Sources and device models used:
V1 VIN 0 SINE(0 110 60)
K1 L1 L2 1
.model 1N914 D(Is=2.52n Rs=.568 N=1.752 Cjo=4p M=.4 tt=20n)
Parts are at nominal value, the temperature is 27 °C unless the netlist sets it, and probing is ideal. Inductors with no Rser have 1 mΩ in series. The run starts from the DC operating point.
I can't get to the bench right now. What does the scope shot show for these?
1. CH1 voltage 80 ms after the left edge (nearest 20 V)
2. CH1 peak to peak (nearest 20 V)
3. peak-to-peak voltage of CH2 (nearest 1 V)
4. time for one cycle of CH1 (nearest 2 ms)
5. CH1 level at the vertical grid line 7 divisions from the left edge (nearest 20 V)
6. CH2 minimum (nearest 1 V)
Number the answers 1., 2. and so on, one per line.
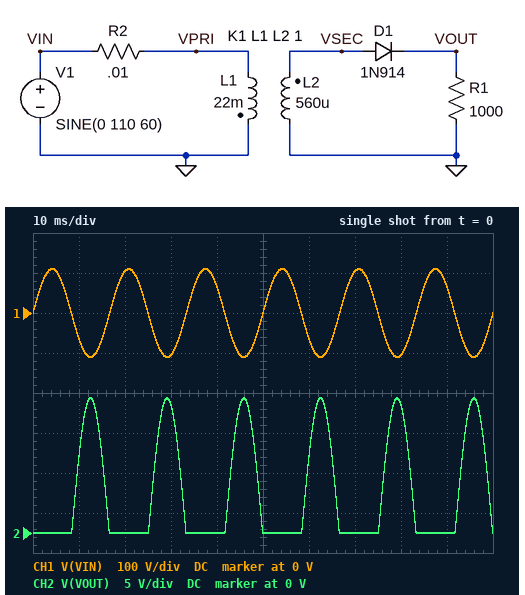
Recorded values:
1. -100 V
2. 220 V
3. 17 V
4. 16 ms
5. 100 V
6. 0 V
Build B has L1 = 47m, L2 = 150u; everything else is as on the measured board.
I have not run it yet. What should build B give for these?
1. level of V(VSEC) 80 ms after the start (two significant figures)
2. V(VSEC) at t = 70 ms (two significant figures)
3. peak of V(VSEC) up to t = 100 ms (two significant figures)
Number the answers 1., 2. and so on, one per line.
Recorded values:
1. 5.9 V
2. -5.9 V
3. 6.2 V
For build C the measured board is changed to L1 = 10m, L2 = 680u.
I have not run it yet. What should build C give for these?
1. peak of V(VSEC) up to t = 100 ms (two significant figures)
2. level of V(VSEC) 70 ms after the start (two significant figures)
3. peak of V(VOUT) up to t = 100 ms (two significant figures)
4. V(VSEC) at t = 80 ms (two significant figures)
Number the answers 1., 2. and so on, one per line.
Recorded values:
1. 29 V
2. -27 V
3. 28 V
4. 27 V
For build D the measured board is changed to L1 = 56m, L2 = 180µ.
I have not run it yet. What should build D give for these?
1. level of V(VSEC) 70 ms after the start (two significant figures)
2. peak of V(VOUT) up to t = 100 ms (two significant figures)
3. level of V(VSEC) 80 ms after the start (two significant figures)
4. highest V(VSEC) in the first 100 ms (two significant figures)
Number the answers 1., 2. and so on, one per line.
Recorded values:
1. -5.9 V
2. 5.6 V
3. 5.9 V
4. 6.2 V
